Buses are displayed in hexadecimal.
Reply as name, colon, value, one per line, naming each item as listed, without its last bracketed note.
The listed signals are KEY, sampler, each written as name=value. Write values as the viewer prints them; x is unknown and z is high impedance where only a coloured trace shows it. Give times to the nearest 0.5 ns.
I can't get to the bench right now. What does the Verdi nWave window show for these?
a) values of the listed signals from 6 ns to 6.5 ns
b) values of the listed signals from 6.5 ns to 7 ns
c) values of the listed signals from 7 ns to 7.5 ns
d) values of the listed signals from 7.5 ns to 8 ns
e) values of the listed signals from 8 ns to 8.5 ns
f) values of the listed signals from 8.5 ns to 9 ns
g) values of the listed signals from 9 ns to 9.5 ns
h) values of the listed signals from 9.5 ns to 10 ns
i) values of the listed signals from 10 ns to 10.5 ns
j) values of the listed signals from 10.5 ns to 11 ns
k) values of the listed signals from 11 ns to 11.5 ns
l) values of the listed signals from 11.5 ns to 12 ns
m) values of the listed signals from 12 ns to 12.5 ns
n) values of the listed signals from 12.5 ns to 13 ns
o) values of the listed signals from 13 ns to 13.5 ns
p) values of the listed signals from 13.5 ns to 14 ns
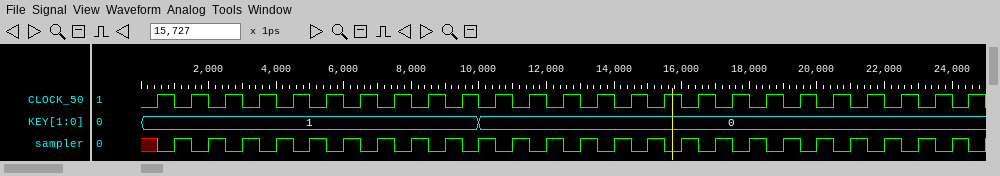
values of the listed signals from 6 ns to 6.5 ns: KEY=1, sampler=1
values of the listed signals from 6.5 ns to 7 ns: KEY=1, sampler=0
values of the listed signals from 7 ns to 7.5 ns: KEY=1, sampler=1
values of the listed signals from 7.5 ns to 8 ns: KEY=1, sampler=0
values of the listed signals from 8 ns to 8.5 ns: KEY=1, sampler=1
values of the listed signals from 8.5 ns to 9 ns: KEY=1, sampler=0
values of the listed signals from 9 ns to 9.5 ns: KEY=1, sampler=1
values of the listed signals from 9.5 ns to 10 ns: KEY=1, sampler=0
values of the listed signals from 10 ns to 10.5 ns: KEY=0, sampler=1
values of the listed signals from 10.5 ns to 11 ns: KEY=0, sampler=0
values of the listed signals from 11 ns to 11.5 ns: KEY=0, sampler=1
values of the listed signals from 11.5 ns to 12 ns: KEY=0, sampler=0
values of the listed signals from 12 ns to 12.5 ns: KEY=0, sampler=1
values of the listed signals from 12.5 ns to 13 ns: KEY=0, sampler=0
values of the listed signals from 13 ns to 13.5 ns: KEY=0, sampler=1
values of the listed signals from 13.5 ns to 14 ns: KEY=0, sampler=0
